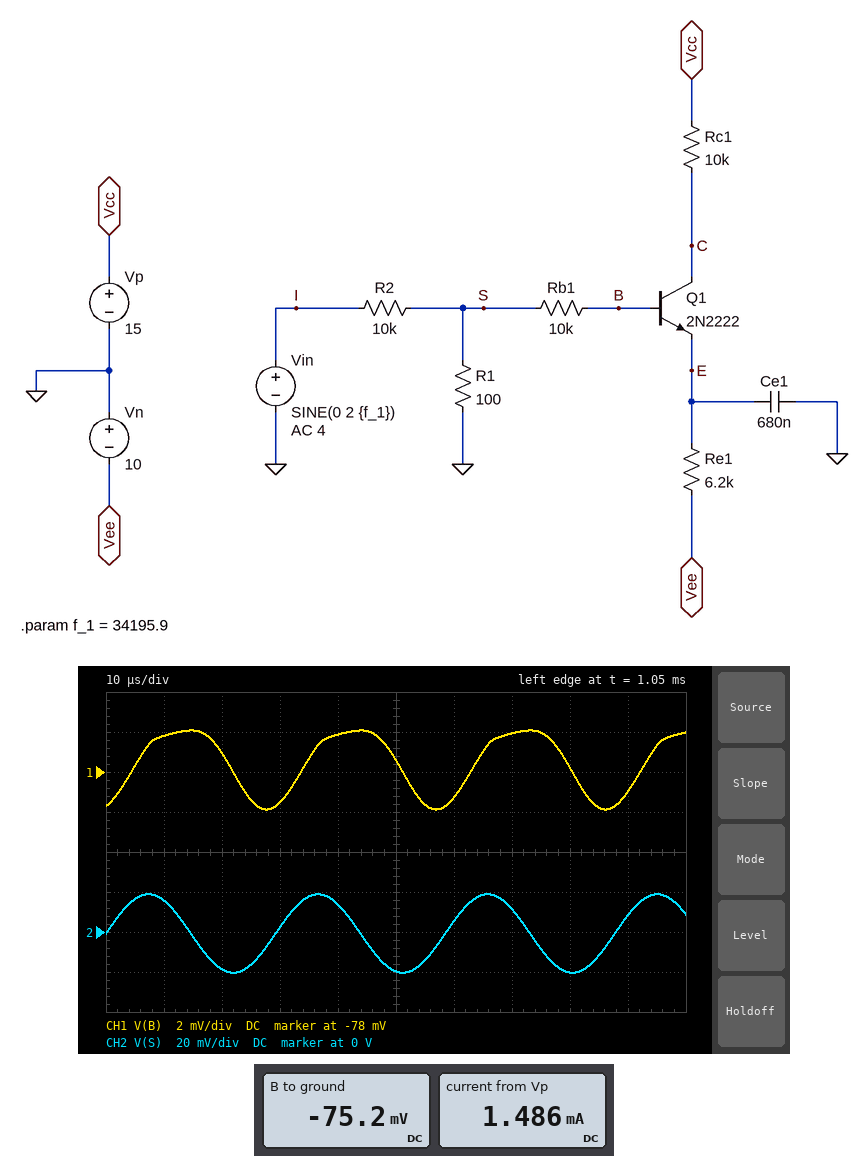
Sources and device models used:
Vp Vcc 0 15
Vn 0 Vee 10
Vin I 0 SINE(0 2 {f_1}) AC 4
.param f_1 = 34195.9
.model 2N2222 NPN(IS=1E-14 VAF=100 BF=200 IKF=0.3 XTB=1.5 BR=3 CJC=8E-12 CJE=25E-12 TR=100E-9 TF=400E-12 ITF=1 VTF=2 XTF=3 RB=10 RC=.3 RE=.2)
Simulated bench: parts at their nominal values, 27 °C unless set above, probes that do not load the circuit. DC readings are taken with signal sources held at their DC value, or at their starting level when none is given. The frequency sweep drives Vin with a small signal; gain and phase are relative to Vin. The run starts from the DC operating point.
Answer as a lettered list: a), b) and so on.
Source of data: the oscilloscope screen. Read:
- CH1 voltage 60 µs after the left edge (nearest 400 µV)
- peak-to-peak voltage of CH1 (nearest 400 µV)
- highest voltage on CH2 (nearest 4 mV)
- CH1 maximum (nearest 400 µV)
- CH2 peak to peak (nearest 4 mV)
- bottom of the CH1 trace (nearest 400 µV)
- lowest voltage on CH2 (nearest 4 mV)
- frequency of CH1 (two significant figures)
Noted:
a) -79.2 mV
b) 4.0 mV
c) 20 mV
d) -76.0 mV
e) 40 mV
f) -80.0 mV
g) -20 mV
h) 34 kHz
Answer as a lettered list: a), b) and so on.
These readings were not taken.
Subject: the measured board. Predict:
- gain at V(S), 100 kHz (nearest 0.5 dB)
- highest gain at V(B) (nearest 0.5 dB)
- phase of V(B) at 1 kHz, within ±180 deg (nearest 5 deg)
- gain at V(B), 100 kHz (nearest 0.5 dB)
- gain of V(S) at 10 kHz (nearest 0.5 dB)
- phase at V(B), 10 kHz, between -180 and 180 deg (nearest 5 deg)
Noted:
a) -40.0 dB
b) -40.0 dB
c) -15 deg
d) -67.5 dB
e) -40.0 dB
f) -65 deg
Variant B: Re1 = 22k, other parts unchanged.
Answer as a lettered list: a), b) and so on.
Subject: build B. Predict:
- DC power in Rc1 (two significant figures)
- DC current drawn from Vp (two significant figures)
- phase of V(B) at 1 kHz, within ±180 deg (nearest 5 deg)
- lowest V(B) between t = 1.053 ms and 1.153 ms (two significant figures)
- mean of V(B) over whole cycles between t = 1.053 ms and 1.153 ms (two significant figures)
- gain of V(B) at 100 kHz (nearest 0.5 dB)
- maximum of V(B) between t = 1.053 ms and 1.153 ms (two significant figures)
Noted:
a) 1.8 mW
b) 420 µA
c) -10 deg
d) -30 mV
e) -19 mV
f) -52.0 dB
g) -10 mV
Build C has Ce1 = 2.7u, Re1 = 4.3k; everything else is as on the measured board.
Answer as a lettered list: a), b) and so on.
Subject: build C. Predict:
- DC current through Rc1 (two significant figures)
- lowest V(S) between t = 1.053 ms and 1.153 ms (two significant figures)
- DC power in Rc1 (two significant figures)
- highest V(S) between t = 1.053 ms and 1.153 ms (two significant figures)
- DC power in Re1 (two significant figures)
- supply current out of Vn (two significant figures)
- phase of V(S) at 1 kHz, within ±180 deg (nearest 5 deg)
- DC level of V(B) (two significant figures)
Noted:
a) 1.7 mA
b) -33 mV
c) 29 mW
d) 5.9 mV
e) 15 mW
f) 1.8 mA
g) 0 deg
h) -1.4 V
